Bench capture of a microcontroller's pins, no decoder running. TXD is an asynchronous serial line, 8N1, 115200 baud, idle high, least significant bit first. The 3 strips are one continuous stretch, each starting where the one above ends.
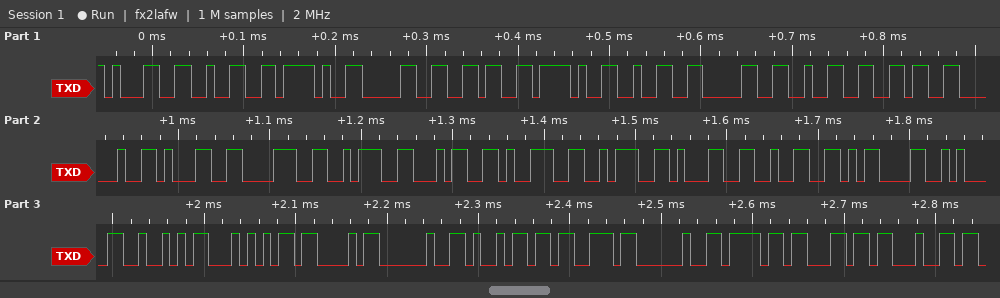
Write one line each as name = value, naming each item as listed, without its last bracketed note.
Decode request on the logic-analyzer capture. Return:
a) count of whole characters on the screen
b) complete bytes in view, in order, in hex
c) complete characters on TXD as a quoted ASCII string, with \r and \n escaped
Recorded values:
count of whole characters on the screen = 31
complete bytes in view, in order, in hex = 0x31 0x32 0x2F 0x30 0x36 0x2F 0x32 0x30 0x32 0x36 0x20 0x31 0x38 0x3A 0x34 0x39 0x3A 0x31 0x32 0x0D 0x0A 0x52 0x54 0x43 0x20 0x69 0x73 0x20 0x6F 0x6C 0x64
complete characters on TXD as a quoted ASCII string, with \r and \n escaped = "12/06/2026 18:49:12\r\nRTC is old"
